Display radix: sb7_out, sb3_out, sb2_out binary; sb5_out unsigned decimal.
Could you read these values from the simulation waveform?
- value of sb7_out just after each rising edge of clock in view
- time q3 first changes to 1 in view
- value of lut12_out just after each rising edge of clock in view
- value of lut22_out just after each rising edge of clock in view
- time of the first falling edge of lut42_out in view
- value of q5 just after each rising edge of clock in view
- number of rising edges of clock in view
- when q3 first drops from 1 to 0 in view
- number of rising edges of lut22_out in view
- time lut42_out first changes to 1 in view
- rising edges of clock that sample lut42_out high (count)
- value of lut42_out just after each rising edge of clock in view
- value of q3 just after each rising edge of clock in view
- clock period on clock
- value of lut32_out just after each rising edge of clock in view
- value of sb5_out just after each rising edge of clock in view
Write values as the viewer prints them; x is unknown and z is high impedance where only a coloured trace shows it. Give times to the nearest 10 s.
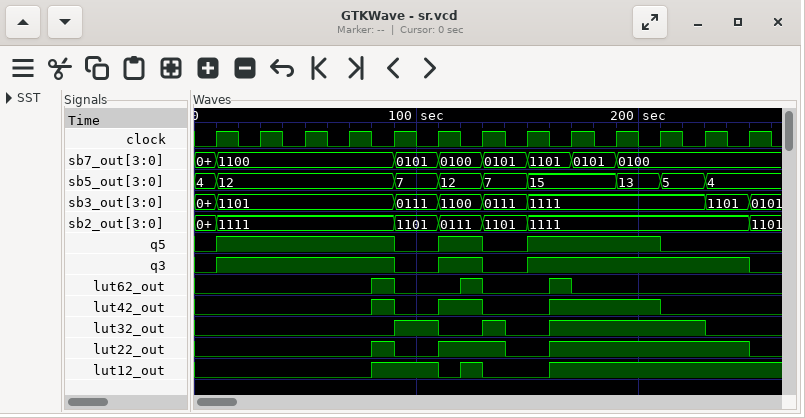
1100, 1100, 1100, 1100, 0101, 0100, 0101, 1101, 0101, 0100, 0100, 0100, 0100
10 s
0 0 0 0 1 0 0 0 1 1 1 1 1
0 0 0 0 0 1 1 0 1 1 1 1 0
90 s
1 1 1 1 0 1 0 1 1 1 0 0 0
13
90 s
3
80 s
5
0 0 0 0 0 1 0 0 1 1 0 0 0
1 1 1 1 0 1 0 1 1 1 1 1 0
20 s
0 0 0 0 1 0 1 0 1 1 1 0 0
12, 12, 12, 12, 7, 12, 7, 15, 15, 13, 5, 4, 4
